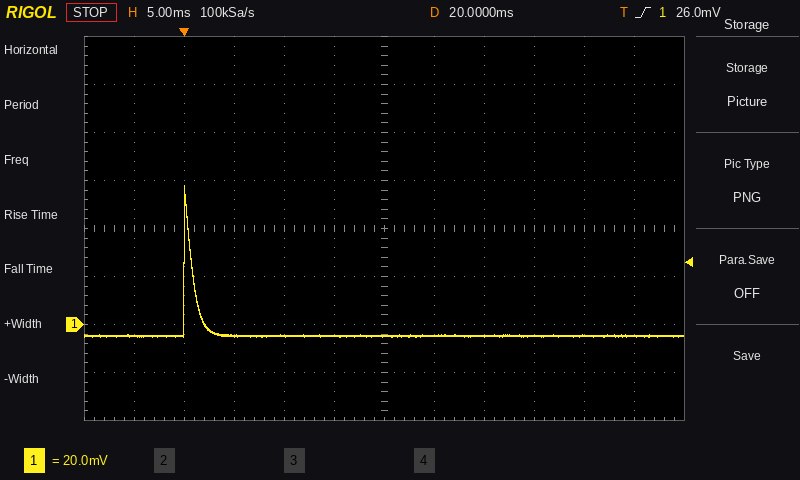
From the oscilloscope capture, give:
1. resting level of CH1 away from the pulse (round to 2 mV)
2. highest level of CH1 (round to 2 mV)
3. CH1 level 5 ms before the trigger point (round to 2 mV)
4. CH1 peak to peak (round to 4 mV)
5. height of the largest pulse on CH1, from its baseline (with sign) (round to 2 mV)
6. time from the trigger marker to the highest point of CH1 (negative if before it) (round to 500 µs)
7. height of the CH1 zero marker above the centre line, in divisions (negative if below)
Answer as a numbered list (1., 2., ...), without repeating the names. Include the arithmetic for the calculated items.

1. -4 mV
2. 58 mV
3. -4 mV
4. 64 mV
5. 58 mV − (-4 mV) = +62 mV
6. 0.0 ms
7. -2.0 div
